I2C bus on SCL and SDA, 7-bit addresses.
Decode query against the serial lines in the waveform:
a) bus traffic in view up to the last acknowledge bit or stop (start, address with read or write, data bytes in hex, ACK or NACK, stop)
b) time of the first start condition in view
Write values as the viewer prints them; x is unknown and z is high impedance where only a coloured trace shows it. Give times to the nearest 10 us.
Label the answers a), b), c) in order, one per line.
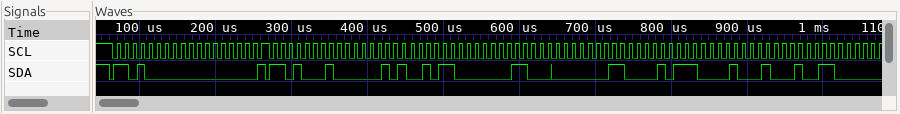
a) start, address 68 write ACK, 00 ACK, repeated start, address 68 read ACK, 05 ACK, 58 ACK, 18 ACK, 03 ACK, 17 ACK, 11 ACK, 26 ACK
b) 60 us
